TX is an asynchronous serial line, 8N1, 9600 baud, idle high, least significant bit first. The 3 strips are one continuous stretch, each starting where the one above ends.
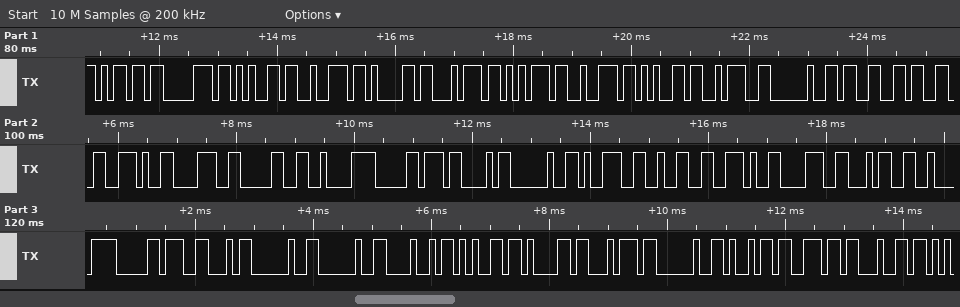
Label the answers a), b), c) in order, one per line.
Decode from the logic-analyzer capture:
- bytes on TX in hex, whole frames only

a) 6D 70 65 72 61 74 75 72 65 3A 20 33 33 2E 38 30 C2 B0 43 20 39 32 2E 38 34 C2 B0 46 20 20 48 65 61 74 20 69 6E 64
